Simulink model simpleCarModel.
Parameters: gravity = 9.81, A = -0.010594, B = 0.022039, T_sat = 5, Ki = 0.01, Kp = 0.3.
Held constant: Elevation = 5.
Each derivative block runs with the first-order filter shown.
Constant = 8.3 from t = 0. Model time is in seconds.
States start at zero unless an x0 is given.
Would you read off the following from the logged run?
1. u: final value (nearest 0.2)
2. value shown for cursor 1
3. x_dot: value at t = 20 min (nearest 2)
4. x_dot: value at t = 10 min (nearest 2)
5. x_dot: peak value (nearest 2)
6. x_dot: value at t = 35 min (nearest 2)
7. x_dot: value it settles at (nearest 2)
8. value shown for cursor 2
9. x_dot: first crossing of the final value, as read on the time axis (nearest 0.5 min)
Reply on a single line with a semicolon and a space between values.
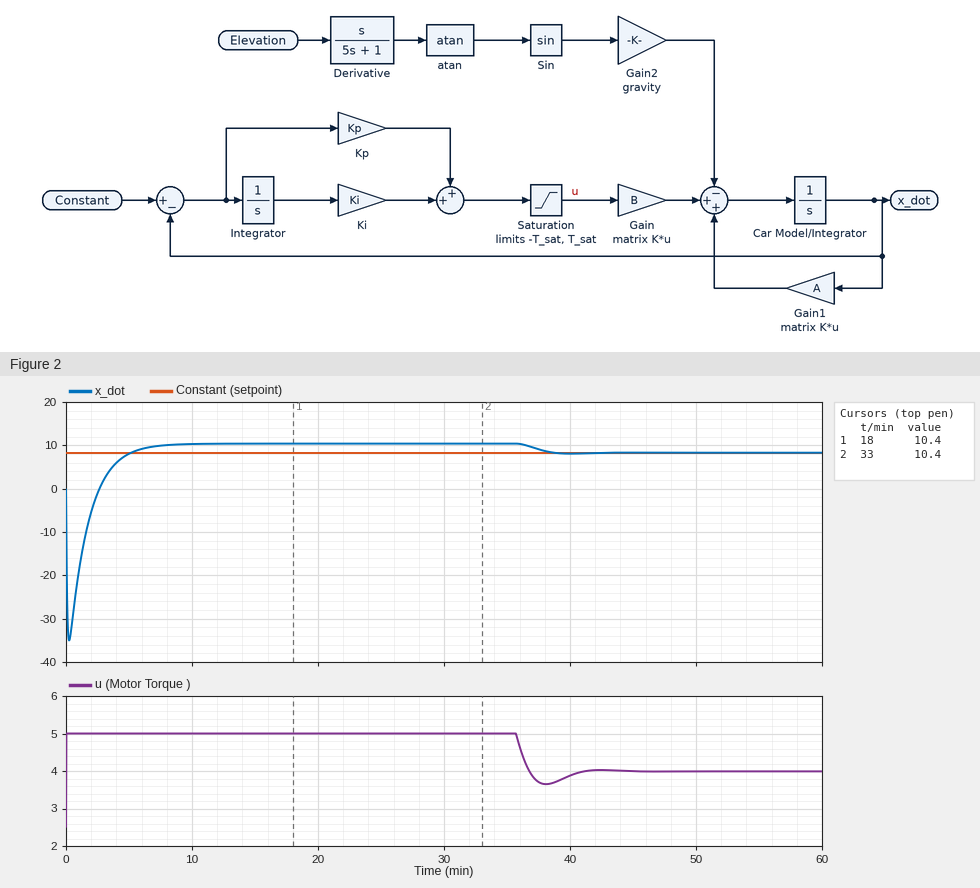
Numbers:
4.0; 10.4; 10; 10; 10; 10; 8; 10.4; 5.0 min
